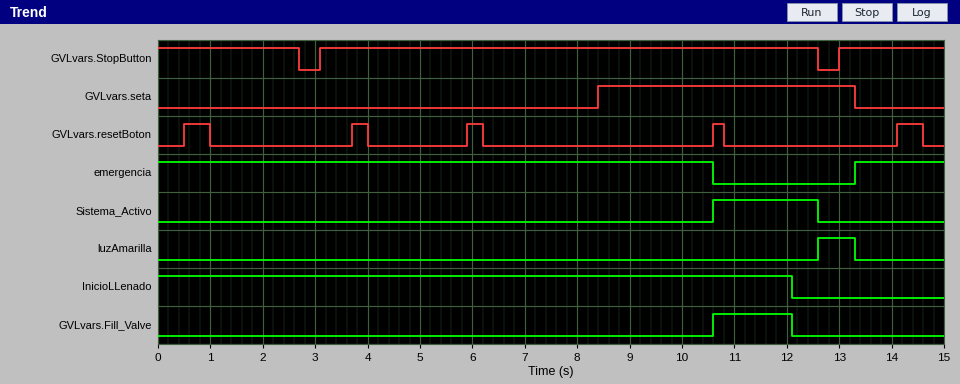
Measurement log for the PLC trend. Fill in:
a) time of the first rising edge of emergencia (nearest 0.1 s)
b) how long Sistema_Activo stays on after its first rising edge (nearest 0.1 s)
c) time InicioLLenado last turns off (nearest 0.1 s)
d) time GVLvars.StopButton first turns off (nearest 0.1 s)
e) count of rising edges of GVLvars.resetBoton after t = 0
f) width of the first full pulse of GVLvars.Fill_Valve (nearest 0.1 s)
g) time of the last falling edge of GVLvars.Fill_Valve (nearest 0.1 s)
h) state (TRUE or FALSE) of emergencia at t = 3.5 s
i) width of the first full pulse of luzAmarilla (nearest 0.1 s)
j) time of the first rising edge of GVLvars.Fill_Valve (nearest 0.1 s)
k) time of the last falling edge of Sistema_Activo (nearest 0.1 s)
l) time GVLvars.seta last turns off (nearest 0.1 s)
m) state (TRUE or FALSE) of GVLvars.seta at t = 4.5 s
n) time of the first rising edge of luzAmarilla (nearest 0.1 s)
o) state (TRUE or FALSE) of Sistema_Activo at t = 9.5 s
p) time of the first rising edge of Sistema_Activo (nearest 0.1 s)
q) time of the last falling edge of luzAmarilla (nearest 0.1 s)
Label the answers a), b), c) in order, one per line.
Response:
a) 13.3 s
b) 2.0 s
c) 12.1 s
d) 2.7 s
e) 5
f) 1.5 s
g) 12.1 s
h) TRUE
i) 0.7 s
j) 10.6 s
k) 12.6 s
l) 13.3 s
m) FALSE
n) 12.6 s
o) FALSE
p) 10.6 s
q) 13.3 s
